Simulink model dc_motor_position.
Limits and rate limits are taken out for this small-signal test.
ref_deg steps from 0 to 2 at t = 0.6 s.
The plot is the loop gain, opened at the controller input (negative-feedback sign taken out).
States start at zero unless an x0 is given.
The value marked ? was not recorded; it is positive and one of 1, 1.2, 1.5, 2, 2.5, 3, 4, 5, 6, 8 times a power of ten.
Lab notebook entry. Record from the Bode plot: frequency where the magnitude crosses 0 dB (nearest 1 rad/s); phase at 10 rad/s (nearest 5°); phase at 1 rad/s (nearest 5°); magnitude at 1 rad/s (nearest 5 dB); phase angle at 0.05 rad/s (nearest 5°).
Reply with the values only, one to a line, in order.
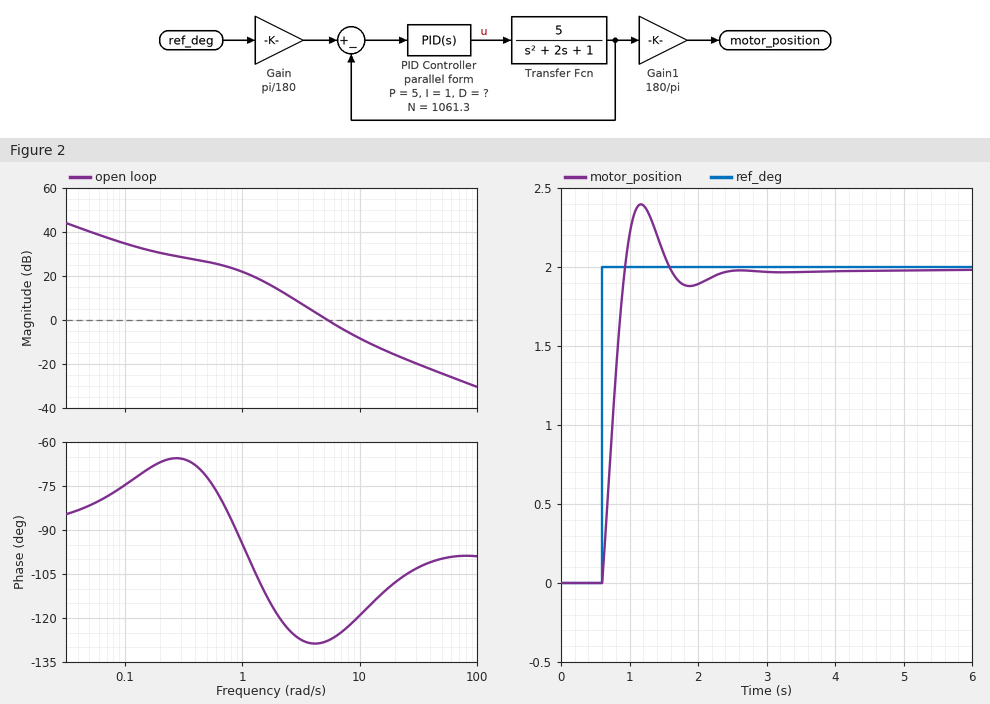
5 rad/s
-120°
-95°
20 dB
-80°
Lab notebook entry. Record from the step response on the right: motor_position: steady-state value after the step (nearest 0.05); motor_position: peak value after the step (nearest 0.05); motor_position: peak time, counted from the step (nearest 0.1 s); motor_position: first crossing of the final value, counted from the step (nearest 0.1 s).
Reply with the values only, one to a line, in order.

2.00
2.40
0.6 s
0.3 s
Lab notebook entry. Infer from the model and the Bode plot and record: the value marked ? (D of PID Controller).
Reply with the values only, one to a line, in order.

0.6
